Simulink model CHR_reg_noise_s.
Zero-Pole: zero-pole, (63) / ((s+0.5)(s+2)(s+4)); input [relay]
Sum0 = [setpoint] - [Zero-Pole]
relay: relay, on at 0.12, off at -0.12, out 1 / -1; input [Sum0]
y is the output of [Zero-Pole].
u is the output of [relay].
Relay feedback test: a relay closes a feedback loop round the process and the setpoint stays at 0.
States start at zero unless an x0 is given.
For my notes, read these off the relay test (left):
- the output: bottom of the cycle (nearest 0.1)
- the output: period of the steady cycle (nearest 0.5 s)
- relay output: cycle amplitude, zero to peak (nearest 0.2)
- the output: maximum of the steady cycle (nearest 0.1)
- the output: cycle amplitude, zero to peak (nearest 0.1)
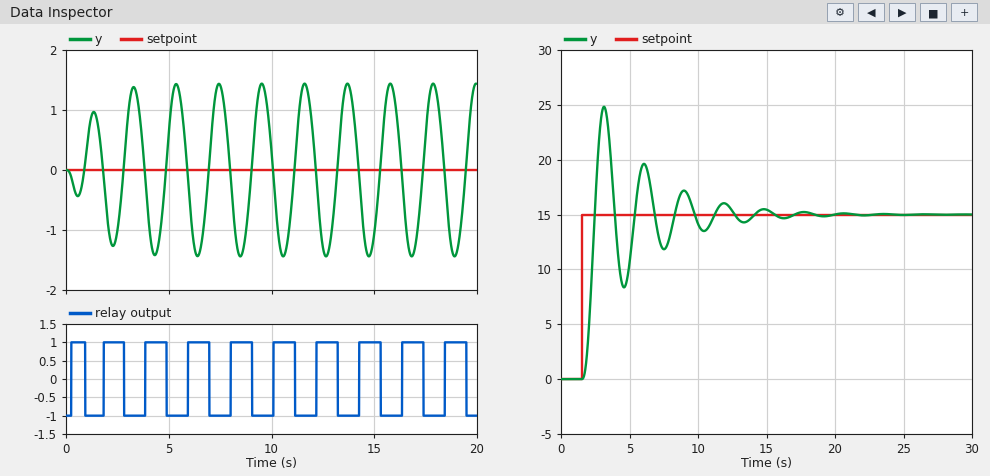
-1.4
2.0 s
1.0
1.4
1.4
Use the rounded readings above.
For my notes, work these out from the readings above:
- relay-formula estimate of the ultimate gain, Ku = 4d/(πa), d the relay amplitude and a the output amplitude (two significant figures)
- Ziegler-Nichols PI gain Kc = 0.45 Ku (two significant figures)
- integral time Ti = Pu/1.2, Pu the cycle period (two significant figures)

0.91
0.41
1.7 s
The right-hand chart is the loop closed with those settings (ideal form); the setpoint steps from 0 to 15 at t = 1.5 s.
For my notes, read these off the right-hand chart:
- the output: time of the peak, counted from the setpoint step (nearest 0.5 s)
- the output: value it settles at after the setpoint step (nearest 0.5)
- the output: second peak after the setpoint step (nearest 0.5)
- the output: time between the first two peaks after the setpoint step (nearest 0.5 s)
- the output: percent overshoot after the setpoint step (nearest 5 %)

1.5 s
15.0
19.5
3.0 s
65 %
